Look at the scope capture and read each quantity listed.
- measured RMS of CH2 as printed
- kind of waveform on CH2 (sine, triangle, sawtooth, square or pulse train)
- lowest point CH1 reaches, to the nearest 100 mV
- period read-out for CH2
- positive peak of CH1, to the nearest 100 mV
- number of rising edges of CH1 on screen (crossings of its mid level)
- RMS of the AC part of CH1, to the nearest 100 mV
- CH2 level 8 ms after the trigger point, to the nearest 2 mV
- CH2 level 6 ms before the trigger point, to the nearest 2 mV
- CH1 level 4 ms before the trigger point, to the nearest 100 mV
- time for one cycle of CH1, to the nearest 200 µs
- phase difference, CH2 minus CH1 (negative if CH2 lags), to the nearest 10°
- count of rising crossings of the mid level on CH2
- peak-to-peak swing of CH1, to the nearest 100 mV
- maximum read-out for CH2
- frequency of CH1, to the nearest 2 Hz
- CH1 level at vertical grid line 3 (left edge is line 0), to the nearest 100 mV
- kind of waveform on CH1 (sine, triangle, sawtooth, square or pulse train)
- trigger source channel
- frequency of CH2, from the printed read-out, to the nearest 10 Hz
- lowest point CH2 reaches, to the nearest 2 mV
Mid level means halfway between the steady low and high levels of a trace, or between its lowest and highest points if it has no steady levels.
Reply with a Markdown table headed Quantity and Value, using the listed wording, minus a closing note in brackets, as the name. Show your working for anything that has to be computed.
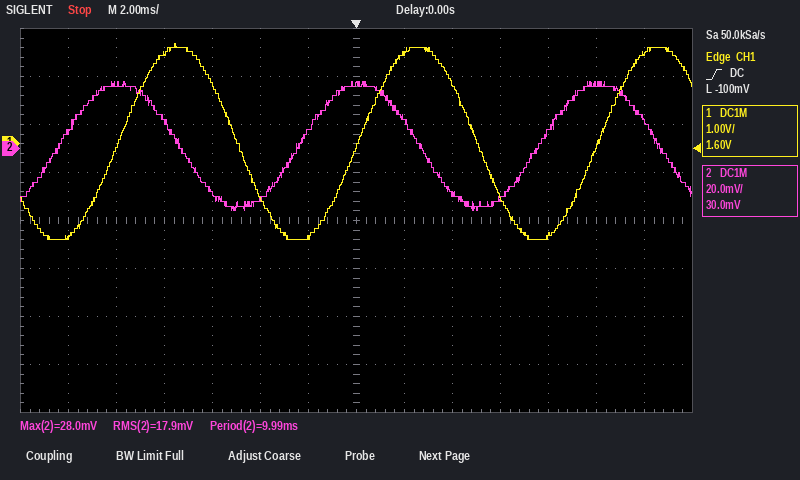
| Quantity | Value |
|---|---|
| measured RMS of CH2 as printed | 17.9 mV |
| kind of waveform on CH2 | sine |
| lowest point CH1 reaches, to the nearest 100 mV | -2.0 V |
| period read-out for CH2 | 9.99 ms |
| positive peak of CH1, to the nearest 100 mV | 2.1 V |
| number of rising edges of CH1 on screen | 3 |
| RMS of the AC part of CH1, to the nearest 100 mV | 4.1 V / (2√2) ≈ 1.4 V |
| CH2 level 8 ms after the trigger point, to the nearest 2 mV | 6 mV |
| CH2 level 6 ms before the trigger point, to the nearest 2 mV | -18 mV |
| CH1 level 4 ms before the trigger point, to the nearest 100 mV | -1.1 V |
| time for one cycle of CH1, to the nearest 200 µs | 10.0 ms |
| phase difference, CH2 minus CH1 (negative if CH2 lags), to the nearest 10° | +90° |
| count of rising crossings of the mid level on CH2 | 3 |
| peak-to-peak swing of CH1, to the nearest 100 mV | 2.1 V − (-2.0 V) = 4.1 V |
| maximum read-out for CH2 | 28.0 mV |
| frequency of CH1, to the nearest 2 Hz | 1 / 10.0 ms ≈ 100 Hz |
| CH1 level at vertical grid line 3 (left edge is line 0), to the nearest 100 mV | 1.9 V |
| kind of waveform on CH1 | sine |
| trigger source channel | CH1 |
| frequency of CH2, from the printed read-out, to the nearest 10 Hz | 1 / 9.99 ms ≈ 100 Hz |
| lowest point CH2 reaches, to the nearest 2 mV | -26 mV |
